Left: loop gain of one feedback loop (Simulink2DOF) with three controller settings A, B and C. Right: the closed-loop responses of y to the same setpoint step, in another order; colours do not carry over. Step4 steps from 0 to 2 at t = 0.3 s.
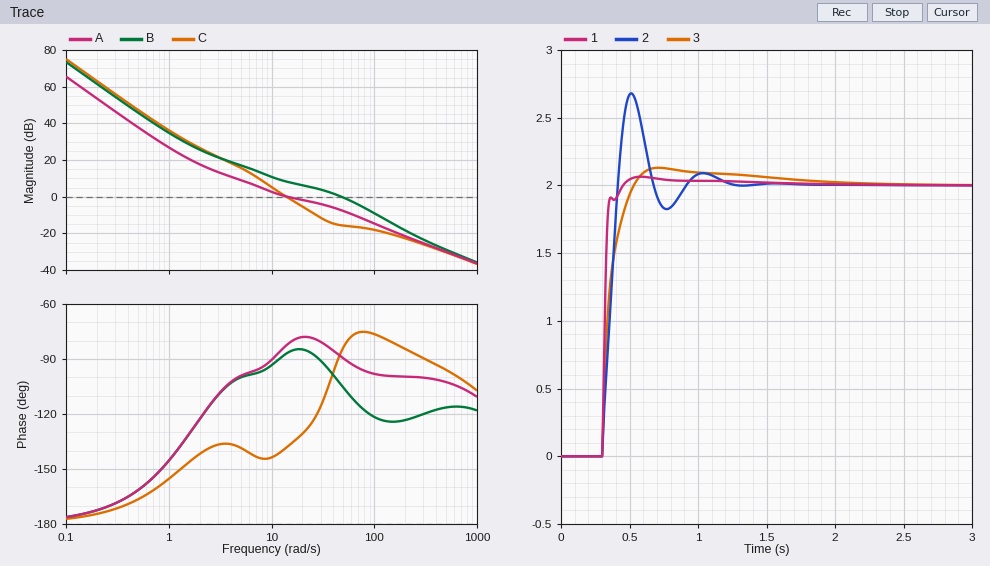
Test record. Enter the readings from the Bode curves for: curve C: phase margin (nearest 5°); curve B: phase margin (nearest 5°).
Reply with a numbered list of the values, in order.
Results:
1. 40°
2. 75°
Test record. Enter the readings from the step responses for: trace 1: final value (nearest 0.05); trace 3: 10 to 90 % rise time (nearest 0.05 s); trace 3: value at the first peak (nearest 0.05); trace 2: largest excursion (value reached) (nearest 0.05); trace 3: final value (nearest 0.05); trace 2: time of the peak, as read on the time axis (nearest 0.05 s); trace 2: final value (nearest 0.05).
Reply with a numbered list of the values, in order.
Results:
1. 2.00
2. 0.15 s
3. 2.15
4. 2.70
5. 2.00
6. 0.50 s
7. 2.00
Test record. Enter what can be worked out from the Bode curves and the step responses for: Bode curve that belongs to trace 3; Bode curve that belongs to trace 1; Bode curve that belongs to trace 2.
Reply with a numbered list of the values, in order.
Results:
1. A
2. B
3. C
